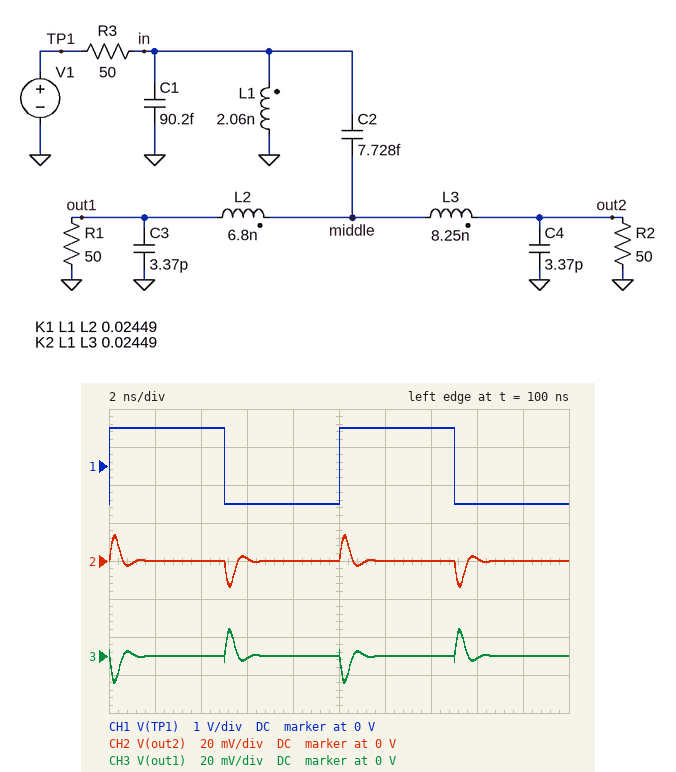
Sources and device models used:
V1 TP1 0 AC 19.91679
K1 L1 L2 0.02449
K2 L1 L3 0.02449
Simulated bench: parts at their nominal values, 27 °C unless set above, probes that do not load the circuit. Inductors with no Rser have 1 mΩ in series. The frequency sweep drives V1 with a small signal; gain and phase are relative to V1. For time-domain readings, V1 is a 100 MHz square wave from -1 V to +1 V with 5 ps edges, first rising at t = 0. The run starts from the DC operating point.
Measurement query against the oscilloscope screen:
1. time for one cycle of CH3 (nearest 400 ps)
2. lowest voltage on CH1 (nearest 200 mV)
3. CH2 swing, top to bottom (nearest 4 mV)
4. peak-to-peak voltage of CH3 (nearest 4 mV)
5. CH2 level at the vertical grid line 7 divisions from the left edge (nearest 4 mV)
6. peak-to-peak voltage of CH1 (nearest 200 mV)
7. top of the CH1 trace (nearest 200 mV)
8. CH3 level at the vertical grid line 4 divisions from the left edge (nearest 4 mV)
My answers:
10.0 ns
-1.0 V
28 mV
28 mV
0 V
2.0 V
1.0 V
0 V
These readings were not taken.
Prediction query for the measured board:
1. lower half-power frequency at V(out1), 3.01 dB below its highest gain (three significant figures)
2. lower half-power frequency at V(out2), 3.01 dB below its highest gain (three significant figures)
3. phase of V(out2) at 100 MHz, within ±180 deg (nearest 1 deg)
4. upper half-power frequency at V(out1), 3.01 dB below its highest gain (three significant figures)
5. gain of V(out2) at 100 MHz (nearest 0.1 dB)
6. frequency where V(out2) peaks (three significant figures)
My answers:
631 MHz
621 MHz
83 deg
1.58 GHz
-58.3 dB
982 MHz
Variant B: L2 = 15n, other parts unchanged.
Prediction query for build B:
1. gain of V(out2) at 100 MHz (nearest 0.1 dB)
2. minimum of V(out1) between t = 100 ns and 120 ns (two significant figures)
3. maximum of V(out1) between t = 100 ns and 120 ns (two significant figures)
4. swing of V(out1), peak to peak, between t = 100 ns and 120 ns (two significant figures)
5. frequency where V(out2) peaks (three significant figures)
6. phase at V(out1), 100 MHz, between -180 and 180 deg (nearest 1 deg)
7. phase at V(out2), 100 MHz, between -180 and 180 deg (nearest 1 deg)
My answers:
-56.5 dB
-12 mV
12 mV
25 mV
785 MHz
-100 deg
80 deg
